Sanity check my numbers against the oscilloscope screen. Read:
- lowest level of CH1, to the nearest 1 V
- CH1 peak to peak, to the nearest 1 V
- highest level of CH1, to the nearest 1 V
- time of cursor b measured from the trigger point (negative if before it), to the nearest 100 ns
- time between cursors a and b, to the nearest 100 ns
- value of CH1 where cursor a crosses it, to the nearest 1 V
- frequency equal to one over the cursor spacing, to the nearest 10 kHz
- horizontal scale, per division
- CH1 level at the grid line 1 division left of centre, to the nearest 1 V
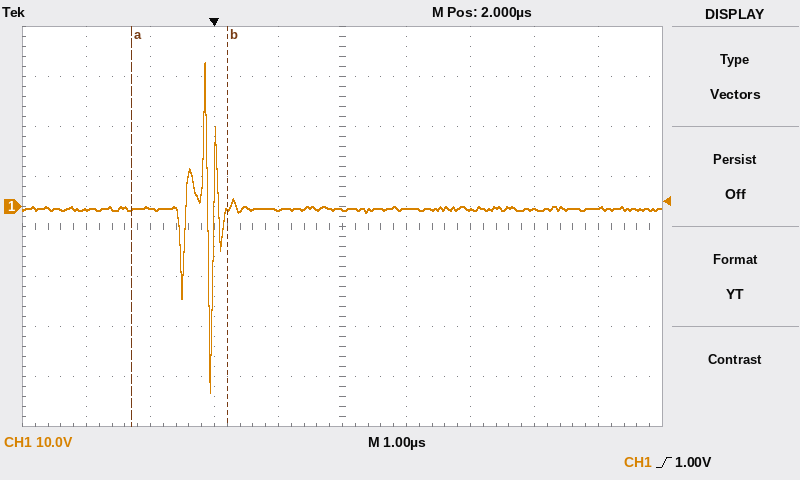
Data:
-37 V
66 V
29 V
+200 ns
1.5 µs
-1 V
670 kHz
1 µs
-1 V
